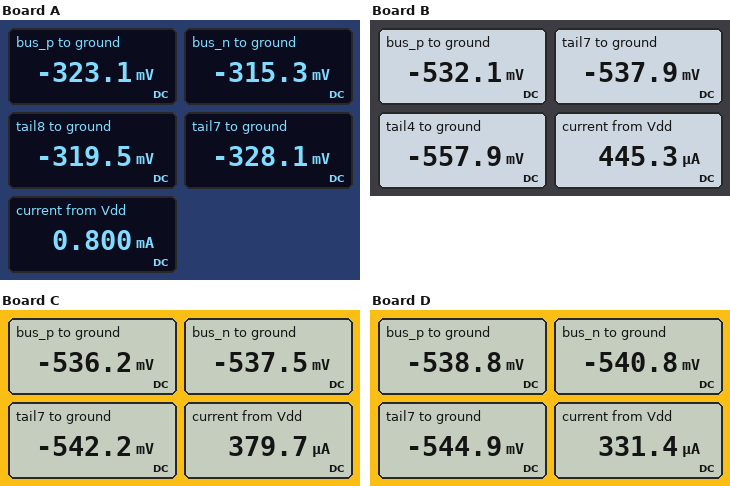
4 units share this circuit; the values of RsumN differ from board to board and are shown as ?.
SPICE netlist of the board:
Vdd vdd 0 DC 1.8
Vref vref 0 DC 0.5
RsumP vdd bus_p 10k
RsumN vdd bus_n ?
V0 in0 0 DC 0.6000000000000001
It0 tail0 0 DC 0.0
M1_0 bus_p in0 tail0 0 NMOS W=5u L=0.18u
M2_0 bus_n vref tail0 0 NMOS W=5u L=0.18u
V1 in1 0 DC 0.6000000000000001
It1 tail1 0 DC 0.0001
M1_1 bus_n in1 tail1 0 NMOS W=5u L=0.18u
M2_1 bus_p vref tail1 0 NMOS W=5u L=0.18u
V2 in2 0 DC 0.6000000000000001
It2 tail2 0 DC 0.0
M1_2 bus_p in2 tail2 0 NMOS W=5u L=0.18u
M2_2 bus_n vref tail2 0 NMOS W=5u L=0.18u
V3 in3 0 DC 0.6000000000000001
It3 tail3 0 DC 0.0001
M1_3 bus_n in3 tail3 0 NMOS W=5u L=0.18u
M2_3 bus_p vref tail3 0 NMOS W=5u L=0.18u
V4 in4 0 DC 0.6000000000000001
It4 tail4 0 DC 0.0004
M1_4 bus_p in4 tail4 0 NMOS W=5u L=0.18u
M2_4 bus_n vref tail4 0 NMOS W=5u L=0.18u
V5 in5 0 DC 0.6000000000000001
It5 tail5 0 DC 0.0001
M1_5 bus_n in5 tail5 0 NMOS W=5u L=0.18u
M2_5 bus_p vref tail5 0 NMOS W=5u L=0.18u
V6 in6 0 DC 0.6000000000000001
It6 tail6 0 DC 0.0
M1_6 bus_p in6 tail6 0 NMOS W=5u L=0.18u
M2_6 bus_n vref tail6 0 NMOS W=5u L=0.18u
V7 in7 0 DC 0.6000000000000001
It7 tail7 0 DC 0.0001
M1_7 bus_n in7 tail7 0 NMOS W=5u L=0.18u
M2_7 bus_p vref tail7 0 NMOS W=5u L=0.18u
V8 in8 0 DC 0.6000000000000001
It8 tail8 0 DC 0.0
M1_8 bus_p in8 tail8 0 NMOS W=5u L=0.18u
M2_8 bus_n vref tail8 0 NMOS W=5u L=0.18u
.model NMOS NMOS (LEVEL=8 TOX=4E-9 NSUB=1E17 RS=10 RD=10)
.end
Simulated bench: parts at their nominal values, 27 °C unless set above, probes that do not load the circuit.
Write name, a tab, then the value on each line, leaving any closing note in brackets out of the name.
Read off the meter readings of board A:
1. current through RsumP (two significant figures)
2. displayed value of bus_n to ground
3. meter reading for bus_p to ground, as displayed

current through RsumP	210 µA
displayed value of bus_n to ground	-315.3 mV
meter reading for bus_p to ground, as displayed	-323.1 mV
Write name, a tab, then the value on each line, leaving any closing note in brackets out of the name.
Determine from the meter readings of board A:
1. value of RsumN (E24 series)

value of RsumN	3.6 kΩ
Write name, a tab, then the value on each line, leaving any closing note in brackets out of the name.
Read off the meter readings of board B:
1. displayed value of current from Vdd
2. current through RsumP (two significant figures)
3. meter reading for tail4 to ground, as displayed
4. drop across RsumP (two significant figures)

displayed value of current from Vdd	445.3 µA
current through RsumP	230 µA
meter reading for tail4 to ground, as displayed	-557.9 mV
drop across RsumP	2.3 V
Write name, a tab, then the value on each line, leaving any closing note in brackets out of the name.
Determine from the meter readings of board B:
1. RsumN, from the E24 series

RsumN, from the E24 series	11 kΩ
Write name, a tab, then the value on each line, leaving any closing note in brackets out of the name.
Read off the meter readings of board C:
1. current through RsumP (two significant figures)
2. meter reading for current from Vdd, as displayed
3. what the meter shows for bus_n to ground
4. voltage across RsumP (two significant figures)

current through RsumP	230 µA
meter reading for current from Vdd, as displayed	379.7 µA
what the meter shows for bus_n to ground	-537.5 mV
voltage across RsumP	2.3 V
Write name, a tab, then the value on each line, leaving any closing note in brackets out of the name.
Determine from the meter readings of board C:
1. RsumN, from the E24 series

RsumN, from the E24 series	16 kΩ
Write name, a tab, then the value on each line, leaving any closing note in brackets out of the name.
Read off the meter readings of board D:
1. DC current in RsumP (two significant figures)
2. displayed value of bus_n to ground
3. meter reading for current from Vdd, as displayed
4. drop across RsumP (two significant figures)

DC current in RsumP	230 µA
displayed value of bus_n to ground	-540.8 mV
meter reading for current from Vdd, as displayed	331.4 µA
drop across RsumP	2.3 V
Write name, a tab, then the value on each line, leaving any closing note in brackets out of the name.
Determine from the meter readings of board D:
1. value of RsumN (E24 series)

value of RsumN	24 kΩ
